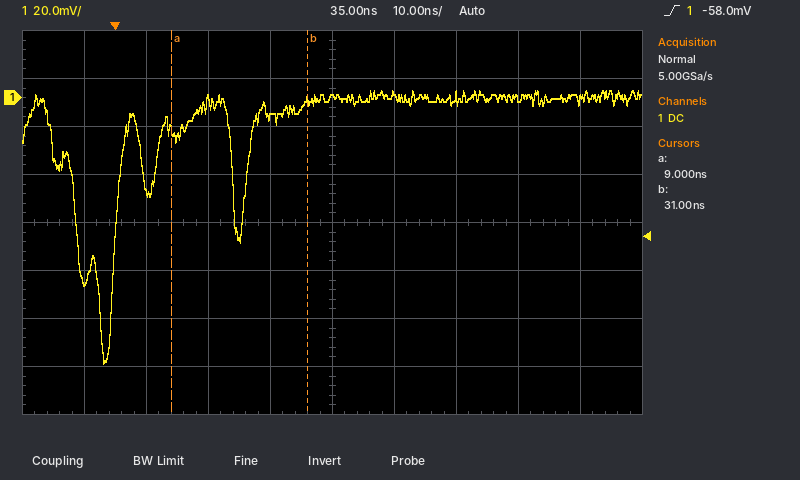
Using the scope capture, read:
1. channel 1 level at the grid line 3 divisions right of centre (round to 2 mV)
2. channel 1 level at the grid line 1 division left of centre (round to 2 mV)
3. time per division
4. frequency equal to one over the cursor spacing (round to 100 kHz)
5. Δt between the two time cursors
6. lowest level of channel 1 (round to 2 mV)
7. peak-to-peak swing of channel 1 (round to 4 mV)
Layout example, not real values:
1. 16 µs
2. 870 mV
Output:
1. 0 mV
2. -8 mV
3. 10 ns
4. 45.5 MHz
5. 22 ns
6. -110 mV
7. 112 mV
